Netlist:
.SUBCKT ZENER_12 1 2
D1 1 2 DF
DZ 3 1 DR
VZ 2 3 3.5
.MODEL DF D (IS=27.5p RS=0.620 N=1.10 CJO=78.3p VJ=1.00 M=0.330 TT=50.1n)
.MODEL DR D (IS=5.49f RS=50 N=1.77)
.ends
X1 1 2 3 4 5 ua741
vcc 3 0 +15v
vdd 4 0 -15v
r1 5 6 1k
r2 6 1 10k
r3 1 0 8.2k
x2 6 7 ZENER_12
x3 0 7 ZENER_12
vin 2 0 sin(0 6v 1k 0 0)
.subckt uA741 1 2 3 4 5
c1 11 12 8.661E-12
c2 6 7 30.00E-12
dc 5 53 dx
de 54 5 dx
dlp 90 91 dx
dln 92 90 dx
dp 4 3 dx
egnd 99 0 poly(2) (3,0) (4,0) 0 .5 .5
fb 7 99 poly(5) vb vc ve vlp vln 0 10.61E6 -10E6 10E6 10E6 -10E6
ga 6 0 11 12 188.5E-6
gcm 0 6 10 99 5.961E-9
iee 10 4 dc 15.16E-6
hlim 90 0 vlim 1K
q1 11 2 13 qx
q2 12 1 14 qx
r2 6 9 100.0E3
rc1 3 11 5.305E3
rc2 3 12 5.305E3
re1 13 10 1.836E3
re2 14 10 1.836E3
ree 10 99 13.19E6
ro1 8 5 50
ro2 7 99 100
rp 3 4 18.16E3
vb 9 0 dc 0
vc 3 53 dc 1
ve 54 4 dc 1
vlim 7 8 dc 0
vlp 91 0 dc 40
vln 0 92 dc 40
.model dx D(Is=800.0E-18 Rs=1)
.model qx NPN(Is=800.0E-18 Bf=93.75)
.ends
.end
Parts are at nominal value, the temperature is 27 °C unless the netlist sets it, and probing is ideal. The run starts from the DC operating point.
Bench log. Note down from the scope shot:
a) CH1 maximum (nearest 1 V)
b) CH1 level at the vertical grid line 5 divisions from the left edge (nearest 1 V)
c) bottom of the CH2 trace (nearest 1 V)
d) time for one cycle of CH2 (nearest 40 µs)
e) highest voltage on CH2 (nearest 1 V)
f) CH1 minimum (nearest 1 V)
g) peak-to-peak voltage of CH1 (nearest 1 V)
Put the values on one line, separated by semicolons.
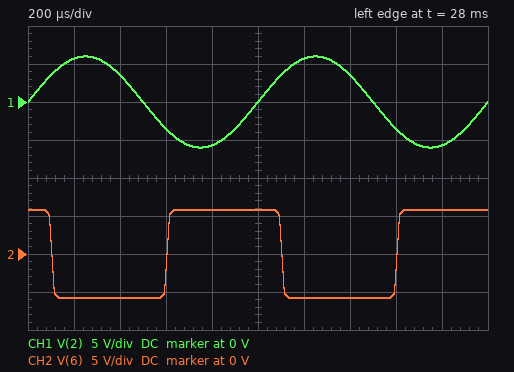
6 V; 0 V; -6 V; 1.00 ms; 6 V; -6 V; 12 V
